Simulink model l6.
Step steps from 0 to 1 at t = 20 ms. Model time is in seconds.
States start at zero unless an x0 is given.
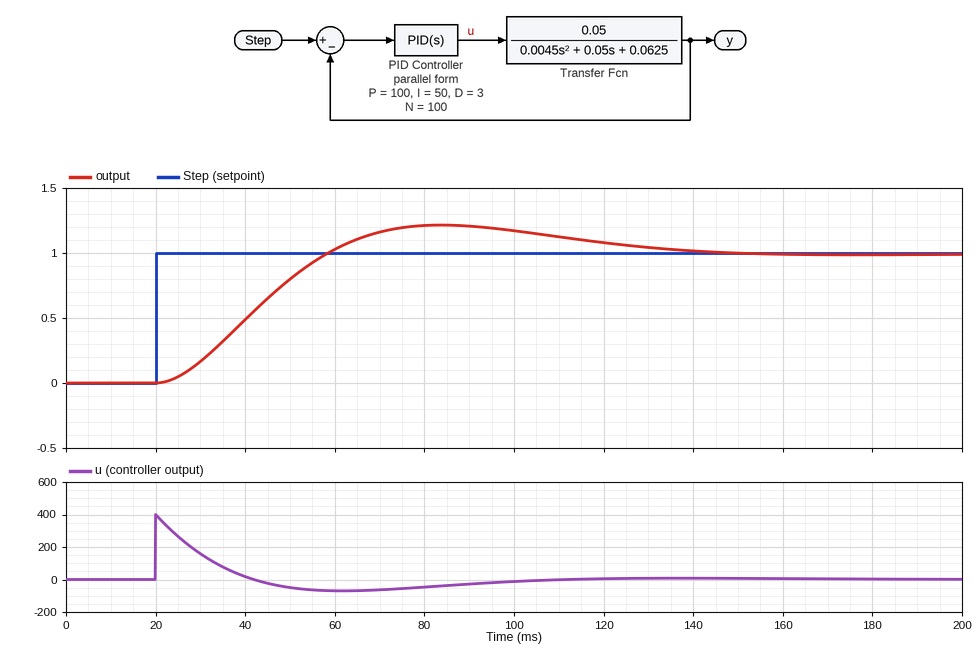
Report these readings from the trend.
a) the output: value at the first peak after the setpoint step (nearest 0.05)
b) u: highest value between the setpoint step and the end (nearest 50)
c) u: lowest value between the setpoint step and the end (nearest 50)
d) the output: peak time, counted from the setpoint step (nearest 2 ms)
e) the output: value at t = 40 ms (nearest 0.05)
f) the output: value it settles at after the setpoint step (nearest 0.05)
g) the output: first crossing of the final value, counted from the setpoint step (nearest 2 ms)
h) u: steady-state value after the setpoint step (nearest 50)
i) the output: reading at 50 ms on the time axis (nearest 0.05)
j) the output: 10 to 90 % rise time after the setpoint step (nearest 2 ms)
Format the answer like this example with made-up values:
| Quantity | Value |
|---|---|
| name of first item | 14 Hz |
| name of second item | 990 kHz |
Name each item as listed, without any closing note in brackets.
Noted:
| Quantity | Value |
|---|---|
| the output: value at the first peak after the setpoint step | 1.20 |
| u: highest value between the setpoint step and the end | 400 |
| u: lowest value between the setpoint step and the end | -50 |
| the output: peak time, counted from the setpoint step | 64 ms |
| the output: value at t = 40 ms | 0.50 |
| the output: value it settles at after the setpoint step | 1.00 |
| the output: first crossing of the final value, counted from the setpoint step | 38 ms |
| u: steady-state value after the setpoint step | 0 |
| the output: reading at 50 ms on the time axis | 0.80 |
| the output: 10 to 90 % rise time after the setpoint step | 26 ms |
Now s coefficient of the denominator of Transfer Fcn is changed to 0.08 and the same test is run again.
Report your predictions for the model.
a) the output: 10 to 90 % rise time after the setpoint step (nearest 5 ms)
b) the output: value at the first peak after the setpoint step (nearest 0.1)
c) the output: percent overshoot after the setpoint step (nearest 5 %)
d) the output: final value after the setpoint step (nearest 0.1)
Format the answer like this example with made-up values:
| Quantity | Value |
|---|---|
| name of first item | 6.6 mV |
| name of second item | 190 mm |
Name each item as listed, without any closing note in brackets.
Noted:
| Quantity | Value |
|---|---|
| the output: 10 to 90 % rise time after the setpoint step | 30 ms |
| the output: value at the first peak after the setpoint step | 1.1 |
| the output: percent overshoot after the setpoint step | 10 % |
| the output: final value after the setpoint step | 1.0 |
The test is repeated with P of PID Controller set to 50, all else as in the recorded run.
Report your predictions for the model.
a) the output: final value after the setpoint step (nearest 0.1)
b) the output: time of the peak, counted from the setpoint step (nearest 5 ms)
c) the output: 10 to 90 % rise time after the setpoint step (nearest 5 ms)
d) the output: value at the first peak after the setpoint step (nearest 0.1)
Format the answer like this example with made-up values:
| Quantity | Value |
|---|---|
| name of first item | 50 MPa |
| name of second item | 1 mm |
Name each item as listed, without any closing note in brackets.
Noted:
| Quantity | Value |
|---|---|
| the output: final value after the setpoint step | 1.0 |
| the output: time of the peak, counted from the setpoint step | 80 ms |
| the output: 10 to 90 % rise time after the setpoint step | 35 ms |
| the output: value at the first peak after the setpoint step | 1.1 |
